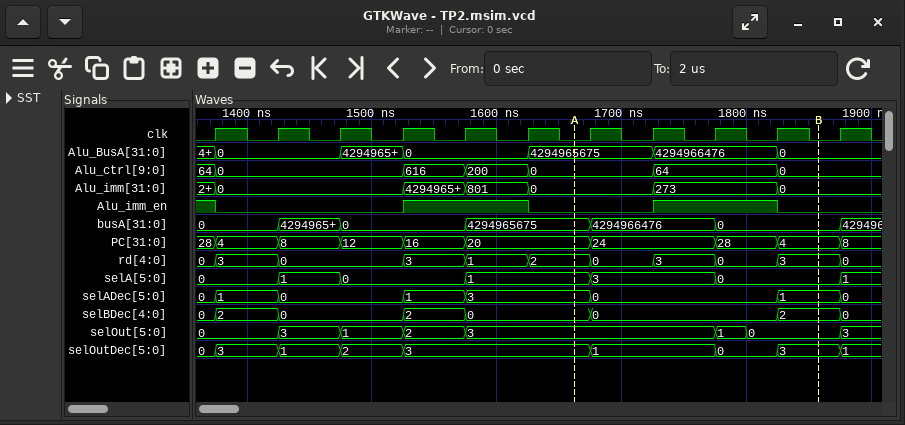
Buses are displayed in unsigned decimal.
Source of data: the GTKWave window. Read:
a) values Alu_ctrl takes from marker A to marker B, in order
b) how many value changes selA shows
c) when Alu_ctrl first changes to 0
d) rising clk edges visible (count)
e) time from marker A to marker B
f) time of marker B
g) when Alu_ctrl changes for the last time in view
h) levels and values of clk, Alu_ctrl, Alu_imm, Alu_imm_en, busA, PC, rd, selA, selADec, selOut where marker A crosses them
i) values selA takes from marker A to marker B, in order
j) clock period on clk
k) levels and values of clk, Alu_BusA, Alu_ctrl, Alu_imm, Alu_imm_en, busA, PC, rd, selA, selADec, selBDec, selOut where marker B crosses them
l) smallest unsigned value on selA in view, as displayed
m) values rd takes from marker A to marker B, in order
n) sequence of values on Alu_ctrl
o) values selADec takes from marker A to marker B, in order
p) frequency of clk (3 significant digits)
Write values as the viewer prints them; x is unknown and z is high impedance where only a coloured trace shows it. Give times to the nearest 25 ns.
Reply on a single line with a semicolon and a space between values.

0, 64, 0; 6; 1375 ns; 11; 200 ns; 1850 ns; 1825 ns; clk=0, Alu_ctrl=0, Alu_imm=0, Alu_imm_en=0, busA=4294965675, PC=20, rd=2, selA=1, selADec=3, selOut=3; 1, 3, 0; 50 ns; clk=0, Alu_BusA=0, Alu_ctrl=0, Alu_imm=0, Alu_imm_en=0, busA=0, PC=4, rd=3, selA=0, selADec=1, selBDec=2, selOut=0; 0; 2, 0, 3, 0, 3; 64, 0, 616, 200, 0, 64, 0; 3, 0, 1; 20.0 MHz
